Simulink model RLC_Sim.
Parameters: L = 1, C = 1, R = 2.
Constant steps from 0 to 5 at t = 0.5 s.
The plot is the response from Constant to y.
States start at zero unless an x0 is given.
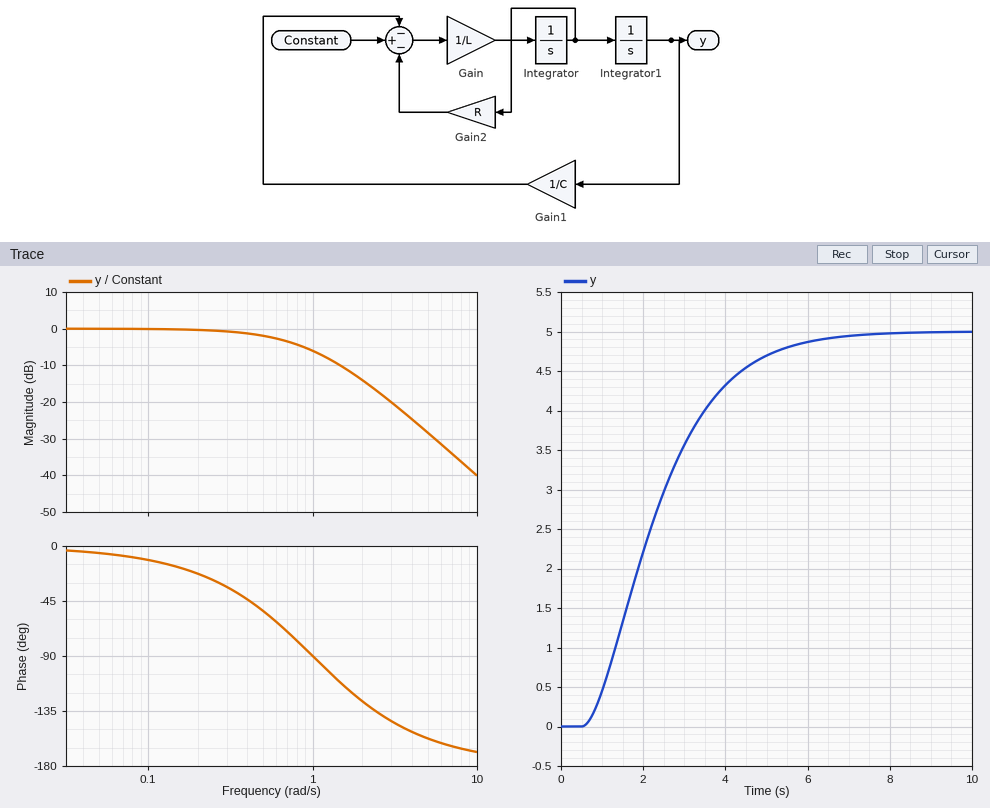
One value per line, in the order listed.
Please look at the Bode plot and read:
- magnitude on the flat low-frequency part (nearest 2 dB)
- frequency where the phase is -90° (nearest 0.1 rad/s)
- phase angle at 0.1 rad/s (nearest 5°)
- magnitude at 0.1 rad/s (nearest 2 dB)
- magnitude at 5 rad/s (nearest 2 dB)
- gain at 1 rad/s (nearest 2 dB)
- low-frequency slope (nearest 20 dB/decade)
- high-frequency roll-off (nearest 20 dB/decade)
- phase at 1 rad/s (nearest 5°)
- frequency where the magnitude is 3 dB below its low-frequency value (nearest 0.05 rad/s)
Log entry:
0 dB
1.0 rad/s
-10°
0 dB
-28 dB
-6 dB
0 dB/decade
-40 dB/decade
-90°
0.65 rad/s
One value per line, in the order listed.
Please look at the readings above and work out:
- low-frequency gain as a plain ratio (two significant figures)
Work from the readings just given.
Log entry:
1.0
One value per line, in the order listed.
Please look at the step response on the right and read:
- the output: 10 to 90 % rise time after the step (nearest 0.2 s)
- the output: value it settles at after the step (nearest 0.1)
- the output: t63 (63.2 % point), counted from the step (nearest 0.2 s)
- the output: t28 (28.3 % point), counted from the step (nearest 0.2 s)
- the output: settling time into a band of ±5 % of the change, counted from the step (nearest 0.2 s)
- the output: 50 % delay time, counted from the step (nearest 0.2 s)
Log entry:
3.4 s
5.0
2.2 s
1.0 s
4.8 s
1.6 s
